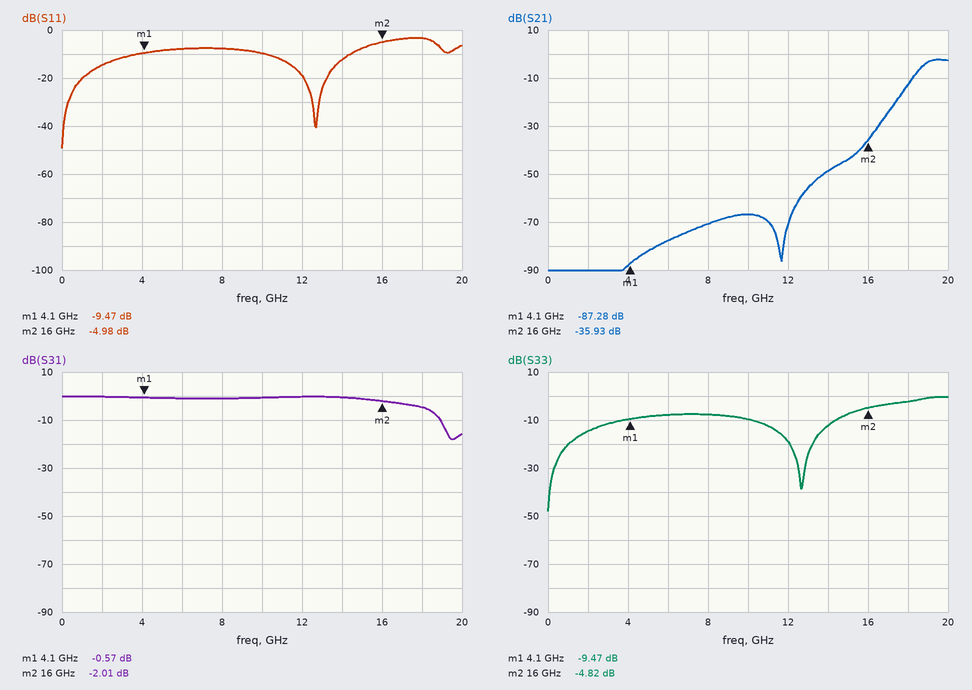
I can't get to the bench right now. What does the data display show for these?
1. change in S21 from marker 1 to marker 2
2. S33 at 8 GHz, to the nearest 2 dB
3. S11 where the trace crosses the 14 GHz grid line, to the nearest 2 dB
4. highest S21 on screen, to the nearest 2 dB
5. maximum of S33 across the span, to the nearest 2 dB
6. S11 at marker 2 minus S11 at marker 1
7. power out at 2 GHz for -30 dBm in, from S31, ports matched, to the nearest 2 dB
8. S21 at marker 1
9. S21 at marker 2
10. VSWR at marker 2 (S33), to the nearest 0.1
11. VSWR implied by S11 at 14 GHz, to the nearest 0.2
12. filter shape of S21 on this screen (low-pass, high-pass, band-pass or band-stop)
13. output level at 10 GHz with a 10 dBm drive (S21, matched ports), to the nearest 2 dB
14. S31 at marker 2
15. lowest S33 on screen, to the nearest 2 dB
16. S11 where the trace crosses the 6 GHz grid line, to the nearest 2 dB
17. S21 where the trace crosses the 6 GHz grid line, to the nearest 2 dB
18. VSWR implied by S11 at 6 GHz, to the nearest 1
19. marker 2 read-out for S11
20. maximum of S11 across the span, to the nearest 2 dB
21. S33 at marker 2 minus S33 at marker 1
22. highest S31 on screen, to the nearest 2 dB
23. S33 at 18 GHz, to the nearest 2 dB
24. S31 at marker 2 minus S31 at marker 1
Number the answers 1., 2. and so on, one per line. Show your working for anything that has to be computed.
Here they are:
1. -35.93 − (-87.28) = 51.35 dB
2. -8 dB
3. -12 dB
4. -2 dB
5. 0 dB
6. -4.98 − (-9.47) = 4.49 dB
7. -30 dBm + (0 dB) = -30 dBm
8. -87.28 dB
9. -35.93 dB
10. (1 + 0.5741)/(1 − 0.5741) ≈ 3.7
11. |Γ| = 10^(-12/20) = 0.2512; VSWR = (1 + 0.2512)/(1 − 0.2512) ≈ 1.67, so 1.6 to the nearest 0.2
12. high-pass
13. 10 dBm + (-66 dB) = -56 dBm
14. -2.01 dB
15. -48 dB
16. -8 dB
17. -78 dB
18. |Γ| = 10^(-8/20) = 0.3981; VSWR = (1 + 0.3981)/(1 − 0.3981) ≈ 2
19. -4.98 dB
20. -4 dB
21. -4.82 − (-9.47) = 4.65 dB
22. 0 dB
23. -2 dB
24. -2.01 − (-0.57) = -1.44 dB
